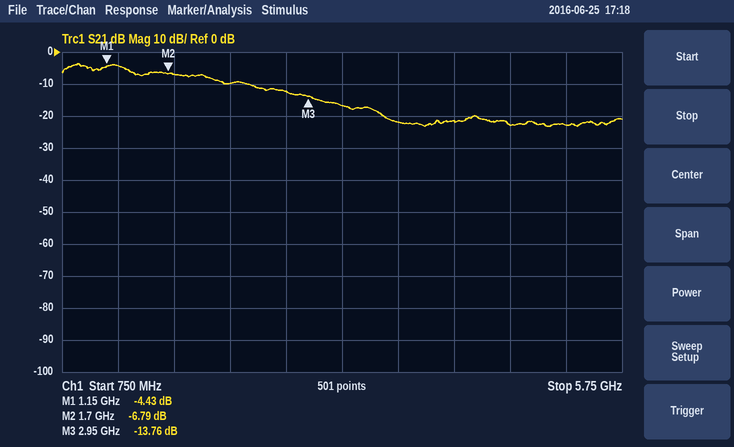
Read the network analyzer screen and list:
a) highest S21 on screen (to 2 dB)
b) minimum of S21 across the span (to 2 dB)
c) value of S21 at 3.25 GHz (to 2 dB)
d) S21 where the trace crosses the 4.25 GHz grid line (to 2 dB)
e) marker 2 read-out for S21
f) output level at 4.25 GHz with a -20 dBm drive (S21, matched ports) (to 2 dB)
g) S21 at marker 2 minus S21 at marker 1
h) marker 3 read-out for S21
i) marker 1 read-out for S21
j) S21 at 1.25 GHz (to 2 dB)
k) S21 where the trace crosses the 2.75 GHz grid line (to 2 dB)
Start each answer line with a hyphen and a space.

- -4 dB
- -24 dB
- -16 dB
- -22 dB
- -6.79 dB
- -42 dBm
- -2.36 dB
- -13.76 dB
- -4.43 dB
- -4 dB
- -12 dB
